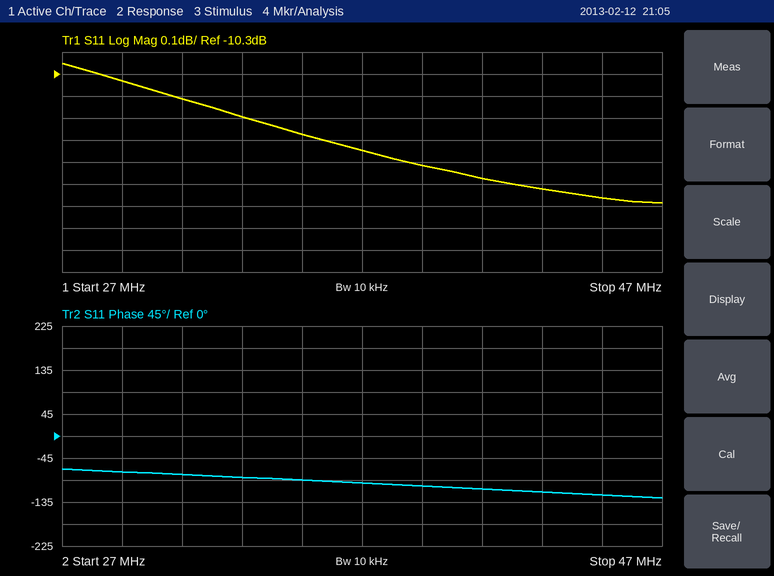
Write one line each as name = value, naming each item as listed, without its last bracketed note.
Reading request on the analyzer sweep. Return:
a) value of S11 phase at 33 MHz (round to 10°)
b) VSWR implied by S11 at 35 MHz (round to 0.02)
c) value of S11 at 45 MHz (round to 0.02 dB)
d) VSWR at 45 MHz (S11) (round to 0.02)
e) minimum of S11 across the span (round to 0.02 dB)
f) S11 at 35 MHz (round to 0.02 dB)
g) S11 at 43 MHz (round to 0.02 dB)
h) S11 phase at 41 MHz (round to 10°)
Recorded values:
value of S11 phase at 33 MHz = -80°
VSWR implied by S11 at 35 MHz = 1.84
value of S11 at 45 MHz = -10.86 dB
VSWR at 45 MHz (S11) = 1.80
minimum of S11 across the span = -10.88 dB
S11 at 35 MHz = -10.58 dB
S11 at 43 MHz = -10.82 dB
S11 phase at 41 MHz = -110°
